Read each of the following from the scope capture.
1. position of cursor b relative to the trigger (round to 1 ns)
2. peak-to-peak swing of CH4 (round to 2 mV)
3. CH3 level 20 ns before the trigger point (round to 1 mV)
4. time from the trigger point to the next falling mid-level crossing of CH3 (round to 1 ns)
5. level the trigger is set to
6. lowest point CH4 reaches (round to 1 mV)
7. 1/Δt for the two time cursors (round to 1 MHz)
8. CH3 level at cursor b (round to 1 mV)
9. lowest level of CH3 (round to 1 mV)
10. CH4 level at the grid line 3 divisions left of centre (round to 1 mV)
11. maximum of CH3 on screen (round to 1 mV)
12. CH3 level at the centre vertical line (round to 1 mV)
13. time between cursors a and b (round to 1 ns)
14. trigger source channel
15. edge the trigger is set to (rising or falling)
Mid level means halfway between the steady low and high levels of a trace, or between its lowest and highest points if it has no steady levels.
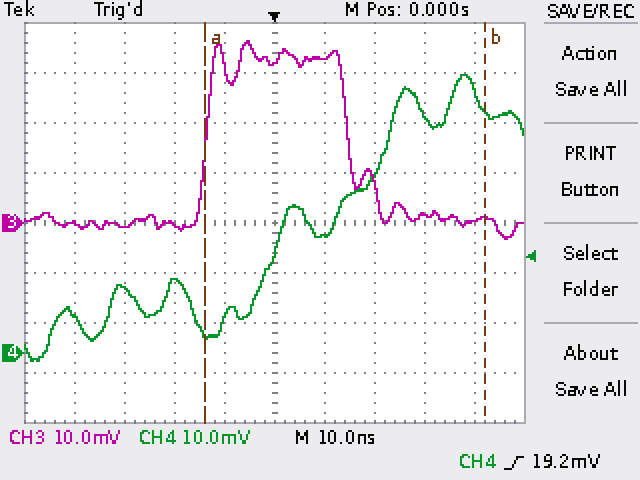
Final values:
+42 ns
58 mV
0 mV
15 ns
19.2 mV
-2 mV
18 MHz
1 mV
-3 mV
13 mV
36 mV
32 mV
56 ns
CH4
rising
